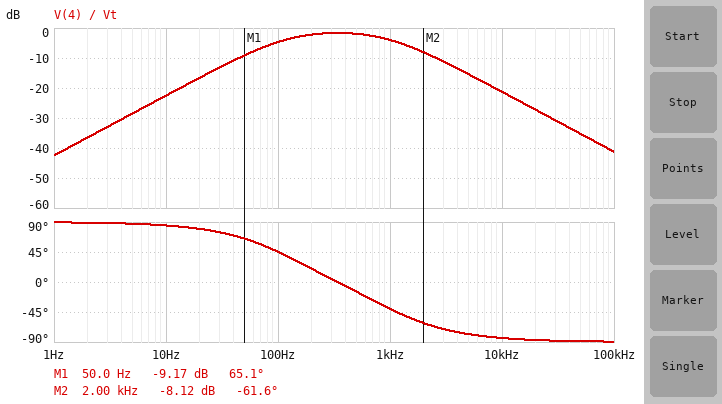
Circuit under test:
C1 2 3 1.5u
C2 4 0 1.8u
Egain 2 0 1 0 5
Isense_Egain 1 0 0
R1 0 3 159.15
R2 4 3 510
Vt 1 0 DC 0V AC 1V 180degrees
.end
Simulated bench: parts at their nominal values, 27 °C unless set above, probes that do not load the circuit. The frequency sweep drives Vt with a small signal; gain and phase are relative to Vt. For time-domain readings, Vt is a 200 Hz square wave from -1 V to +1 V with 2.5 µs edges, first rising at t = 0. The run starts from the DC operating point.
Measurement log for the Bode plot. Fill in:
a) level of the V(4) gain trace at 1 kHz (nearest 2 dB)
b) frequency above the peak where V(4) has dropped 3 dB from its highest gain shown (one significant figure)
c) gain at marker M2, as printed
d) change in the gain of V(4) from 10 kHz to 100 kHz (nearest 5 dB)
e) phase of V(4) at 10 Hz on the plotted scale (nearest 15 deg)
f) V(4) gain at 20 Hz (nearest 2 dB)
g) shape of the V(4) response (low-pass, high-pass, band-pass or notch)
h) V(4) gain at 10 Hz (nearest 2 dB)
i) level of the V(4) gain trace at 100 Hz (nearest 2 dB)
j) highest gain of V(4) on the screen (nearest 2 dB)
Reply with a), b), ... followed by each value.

a) -4 dB
b) 1 kHz
c) -8.12 dB
d) -20 dB
e) 90 deg
f) -16 dB
g) band-pass
h) -22 dB
i) -4 dB
j) -2 dB
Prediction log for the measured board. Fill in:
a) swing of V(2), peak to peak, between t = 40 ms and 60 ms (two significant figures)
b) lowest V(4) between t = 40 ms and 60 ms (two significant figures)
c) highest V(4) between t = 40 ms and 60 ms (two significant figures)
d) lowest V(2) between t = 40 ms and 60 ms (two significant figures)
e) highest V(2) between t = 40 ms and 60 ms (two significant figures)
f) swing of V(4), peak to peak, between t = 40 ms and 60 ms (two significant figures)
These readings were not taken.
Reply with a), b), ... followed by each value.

a) 10 V
b) -1.2 V
c) 1.2 V
d) -5.0 V
e) 5.0 V
f) 2.4 V
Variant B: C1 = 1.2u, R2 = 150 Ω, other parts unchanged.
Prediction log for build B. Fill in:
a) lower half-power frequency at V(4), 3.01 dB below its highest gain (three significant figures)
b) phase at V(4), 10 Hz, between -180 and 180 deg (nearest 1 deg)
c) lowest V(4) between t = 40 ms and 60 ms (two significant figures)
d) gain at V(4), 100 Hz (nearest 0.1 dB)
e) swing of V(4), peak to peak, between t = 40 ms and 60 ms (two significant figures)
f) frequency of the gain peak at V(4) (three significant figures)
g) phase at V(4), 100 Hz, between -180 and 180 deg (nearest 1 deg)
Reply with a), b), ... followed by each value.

a) 196 Hz
b) 87 deg
c) -2.1 V
d) -5.2 dB
e) 4.2 V
f) 701 Hz
g) 64 deg
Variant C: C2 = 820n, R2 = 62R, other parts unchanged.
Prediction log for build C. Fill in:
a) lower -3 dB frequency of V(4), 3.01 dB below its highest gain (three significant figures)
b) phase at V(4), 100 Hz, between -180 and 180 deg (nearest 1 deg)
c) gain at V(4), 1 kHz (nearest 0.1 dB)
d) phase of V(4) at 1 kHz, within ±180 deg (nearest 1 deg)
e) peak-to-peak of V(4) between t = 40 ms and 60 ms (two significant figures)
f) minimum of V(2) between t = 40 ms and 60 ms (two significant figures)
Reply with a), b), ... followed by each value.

a) 356 Hz
b) 75 deg
c) 8.9 dB
d) 11 deg
e) 9.9 V
f) -5.0 V
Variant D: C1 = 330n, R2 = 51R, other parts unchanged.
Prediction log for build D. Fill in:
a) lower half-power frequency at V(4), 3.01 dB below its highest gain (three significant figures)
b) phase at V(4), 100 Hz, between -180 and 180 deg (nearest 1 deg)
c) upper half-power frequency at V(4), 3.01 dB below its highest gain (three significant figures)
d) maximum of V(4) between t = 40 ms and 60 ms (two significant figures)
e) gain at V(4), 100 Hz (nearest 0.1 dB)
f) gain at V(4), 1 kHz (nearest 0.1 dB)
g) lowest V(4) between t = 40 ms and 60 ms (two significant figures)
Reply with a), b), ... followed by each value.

a) 360 Hz
b) 75 deg
c) 14.6 kHz
d) 1.1 V
e) -15.9 dB
f) -4.7 dB
g) -1.1 V
